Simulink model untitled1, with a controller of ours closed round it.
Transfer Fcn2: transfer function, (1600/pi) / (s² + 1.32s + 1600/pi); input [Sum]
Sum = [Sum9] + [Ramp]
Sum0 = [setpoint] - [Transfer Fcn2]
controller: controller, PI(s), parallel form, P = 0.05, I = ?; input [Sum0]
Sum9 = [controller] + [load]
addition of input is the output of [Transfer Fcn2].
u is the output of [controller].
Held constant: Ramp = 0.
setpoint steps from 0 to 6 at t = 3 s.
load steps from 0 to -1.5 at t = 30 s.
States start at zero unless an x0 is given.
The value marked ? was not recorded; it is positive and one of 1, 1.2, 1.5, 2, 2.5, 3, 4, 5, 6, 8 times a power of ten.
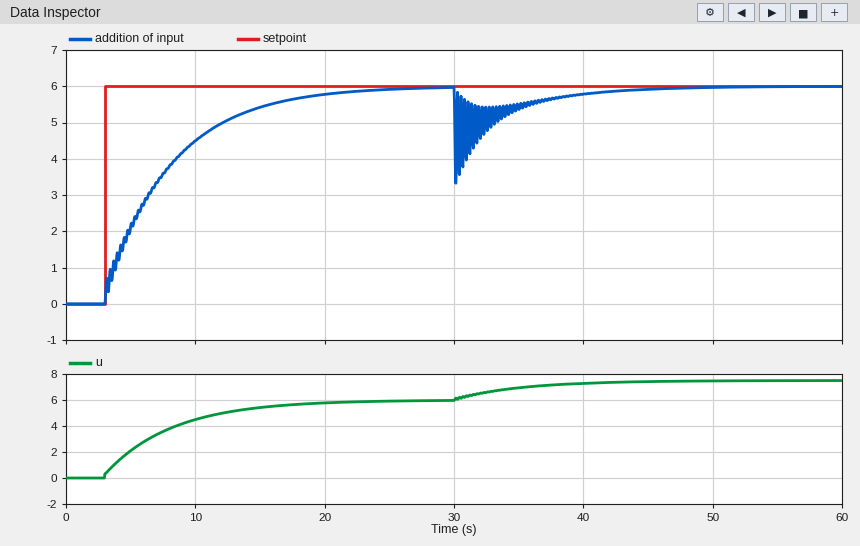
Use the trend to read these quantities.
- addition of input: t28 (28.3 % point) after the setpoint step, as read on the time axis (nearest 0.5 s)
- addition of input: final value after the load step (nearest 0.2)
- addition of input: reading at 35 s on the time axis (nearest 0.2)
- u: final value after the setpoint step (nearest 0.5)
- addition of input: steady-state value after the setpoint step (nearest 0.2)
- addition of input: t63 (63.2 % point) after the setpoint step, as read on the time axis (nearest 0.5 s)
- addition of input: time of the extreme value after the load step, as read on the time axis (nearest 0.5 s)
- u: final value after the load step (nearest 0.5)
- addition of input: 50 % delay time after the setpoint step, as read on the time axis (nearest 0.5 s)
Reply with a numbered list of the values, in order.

1. 4.5 s
2. 6.0
3. 5.4
4. 6.0
5. 6.0
6. 8.0 s
7. 30.0 s
8. 7.5
9. 6.5 s
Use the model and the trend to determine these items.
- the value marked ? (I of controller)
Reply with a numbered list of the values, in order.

1. 0.2
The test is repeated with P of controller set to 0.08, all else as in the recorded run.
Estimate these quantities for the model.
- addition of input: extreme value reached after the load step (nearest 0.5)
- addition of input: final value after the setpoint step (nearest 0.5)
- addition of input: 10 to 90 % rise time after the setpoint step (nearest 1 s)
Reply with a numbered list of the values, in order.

1. 3.5
2. 6.0
3. 12 s
